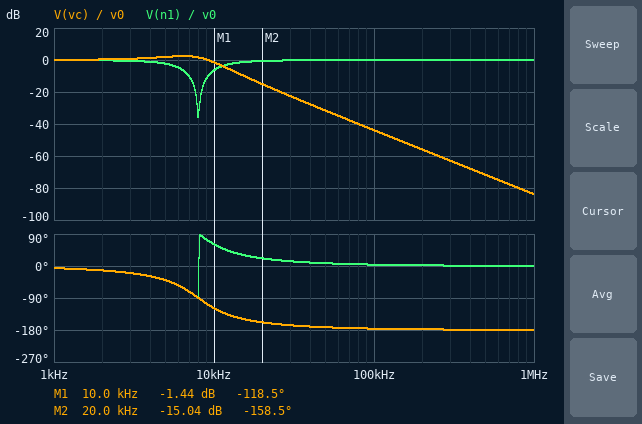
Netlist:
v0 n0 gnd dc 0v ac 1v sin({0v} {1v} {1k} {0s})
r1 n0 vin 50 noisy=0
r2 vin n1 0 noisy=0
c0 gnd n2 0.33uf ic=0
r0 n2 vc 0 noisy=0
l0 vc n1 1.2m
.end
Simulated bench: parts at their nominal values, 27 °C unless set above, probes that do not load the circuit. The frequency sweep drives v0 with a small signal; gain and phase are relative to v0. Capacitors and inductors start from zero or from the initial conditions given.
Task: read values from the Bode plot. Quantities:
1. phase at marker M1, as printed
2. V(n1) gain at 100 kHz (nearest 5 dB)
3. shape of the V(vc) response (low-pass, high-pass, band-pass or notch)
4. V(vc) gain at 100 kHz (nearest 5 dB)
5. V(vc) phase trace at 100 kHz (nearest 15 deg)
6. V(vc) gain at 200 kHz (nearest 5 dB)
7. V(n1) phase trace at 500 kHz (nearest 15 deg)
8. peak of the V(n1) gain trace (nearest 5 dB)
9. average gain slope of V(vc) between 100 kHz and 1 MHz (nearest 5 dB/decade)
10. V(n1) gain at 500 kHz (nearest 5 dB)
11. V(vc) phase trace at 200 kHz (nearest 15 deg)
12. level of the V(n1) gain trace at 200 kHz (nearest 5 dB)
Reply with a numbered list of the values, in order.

1. -118.5 deg
2. 0 dB
3. low-pass
4. -45 dB
5. -180 deg
6. -55 dB
7. 0 deg
8. 0 dB
9. -40 dB/decade
10. 0 dB
11. -180 deg
12. 0 dB
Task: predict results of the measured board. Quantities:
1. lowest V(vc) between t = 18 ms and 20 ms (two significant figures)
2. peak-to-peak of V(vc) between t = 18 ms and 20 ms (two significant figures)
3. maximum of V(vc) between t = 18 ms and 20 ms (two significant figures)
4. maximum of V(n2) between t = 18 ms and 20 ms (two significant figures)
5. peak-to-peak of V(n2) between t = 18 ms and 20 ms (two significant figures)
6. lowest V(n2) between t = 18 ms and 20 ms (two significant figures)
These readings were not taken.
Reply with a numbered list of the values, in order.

1. -1.0 V
2. 2.0 V
3. 1.0 V
4. 1.0 V
5. 2.0 V
6. -1.0 V
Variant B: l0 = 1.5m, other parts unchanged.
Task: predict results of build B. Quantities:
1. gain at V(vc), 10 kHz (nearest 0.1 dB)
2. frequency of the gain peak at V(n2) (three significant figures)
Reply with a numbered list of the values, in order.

1. -3.0 dB
2. 6.09 kHz
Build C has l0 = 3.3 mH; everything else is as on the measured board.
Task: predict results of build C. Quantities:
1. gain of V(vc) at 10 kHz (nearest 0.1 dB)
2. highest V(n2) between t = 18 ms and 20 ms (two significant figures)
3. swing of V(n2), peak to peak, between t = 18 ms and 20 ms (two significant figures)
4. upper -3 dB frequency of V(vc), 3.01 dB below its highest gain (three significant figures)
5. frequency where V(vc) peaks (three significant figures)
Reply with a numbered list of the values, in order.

1. -10.8 dB
2. 1.0 V
3. 2.1 V
4. 5.62 kHz
5. 4.51 kHz
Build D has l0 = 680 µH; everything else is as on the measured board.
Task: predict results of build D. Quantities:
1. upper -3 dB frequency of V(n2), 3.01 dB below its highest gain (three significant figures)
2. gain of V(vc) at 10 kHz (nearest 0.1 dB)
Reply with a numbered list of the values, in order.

1. 12.2 kHz
2. -0.4 dB
